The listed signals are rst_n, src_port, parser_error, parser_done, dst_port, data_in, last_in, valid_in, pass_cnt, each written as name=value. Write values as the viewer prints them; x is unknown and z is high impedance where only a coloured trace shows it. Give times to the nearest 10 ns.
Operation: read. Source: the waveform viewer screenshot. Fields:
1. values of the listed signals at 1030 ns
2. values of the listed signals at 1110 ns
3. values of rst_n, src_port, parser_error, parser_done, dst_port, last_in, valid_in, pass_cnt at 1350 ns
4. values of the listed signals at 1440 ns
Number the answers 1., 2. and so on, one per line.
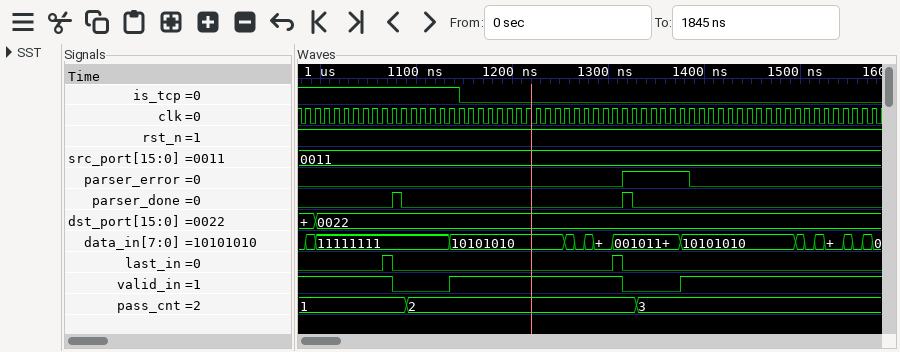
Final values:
1. rst_n=1, src_port=0011, parser_error=0, parser_done=0, dst_port=0022, data_in=11111111, last_in=0, valid_in=1, pass_cnt=1
2. rst_n=1, src_port=0011, parser_error=0, parser_done=0, dst_port=0022, data_in=11111111, last_in=0, valid_in=0, pass_cnt=2
3. rst_n=1, src_port=0011, parser_error=1, parser_done=0, dst_port=0022, last_in=0, valid_in=0, pass_cnt=3
4. rst_n=1, src_port=0011, parser_error=0, parser_done=0, dst_port=0022, data_in=10101010, last_in=0, valid_in=1, pass_cnt=3
